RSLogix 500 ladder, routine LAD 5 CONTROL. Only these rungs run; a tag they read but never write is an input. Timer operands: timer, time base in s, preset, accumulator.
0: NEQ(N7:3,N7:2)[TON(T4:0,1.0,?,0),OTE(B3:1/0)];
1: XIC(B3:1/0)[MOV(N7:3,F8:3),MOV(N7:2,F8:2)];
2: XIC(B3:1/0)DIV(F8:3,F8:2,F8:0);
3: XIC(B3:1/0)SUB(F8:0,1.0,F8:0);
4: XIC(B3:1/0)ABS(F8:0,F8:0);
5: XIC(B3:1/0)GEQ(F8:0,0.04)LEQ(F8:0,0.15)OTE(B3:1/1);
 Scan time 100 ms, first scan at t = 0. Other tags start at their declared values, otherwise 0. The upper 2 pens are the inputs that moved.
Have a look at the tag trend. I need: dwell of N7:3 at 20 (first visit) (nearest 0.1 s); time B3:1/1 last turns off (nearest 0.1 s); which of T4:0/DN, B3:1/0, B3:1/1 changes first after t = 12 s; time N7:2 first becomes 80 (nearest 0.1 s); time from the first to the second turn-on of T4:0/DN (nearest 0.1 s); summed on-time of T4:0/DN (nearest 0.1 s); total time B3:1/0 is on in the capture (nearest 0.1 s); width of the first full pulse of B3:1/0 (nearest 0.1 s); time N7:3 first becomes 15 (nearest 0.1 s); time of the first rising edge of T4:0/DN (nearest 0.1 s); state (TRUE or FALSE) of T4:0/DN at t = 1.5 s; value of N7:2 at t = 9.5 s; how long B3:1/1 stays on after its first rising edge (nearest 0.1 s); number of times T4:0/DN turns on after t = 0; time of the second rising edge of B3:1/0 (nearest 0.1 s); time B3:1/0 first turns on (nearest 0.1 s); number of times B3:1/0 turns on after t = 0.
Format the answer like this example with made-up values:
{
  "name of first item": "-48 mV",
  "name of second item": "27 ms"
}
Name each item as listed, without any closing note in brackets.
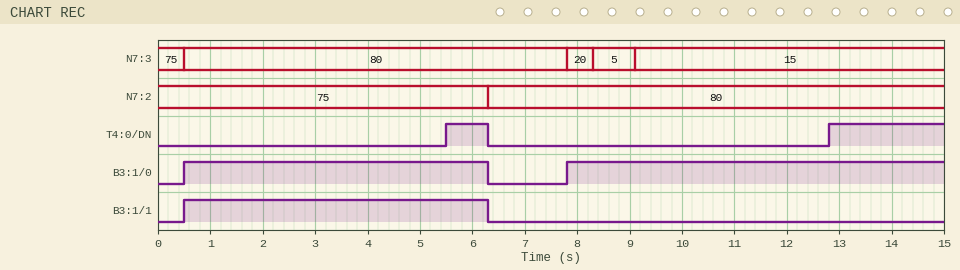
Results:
{
  "dwell of N7:3 at 20 (first visit)": "0.5 s",
  "time B3:1/1 last turns off": "6.3 s",
  "which of T4:0/DN, B3:1/0, B3:1/1 changes first after t = 12 s": "T4:0/DN",
  "time N7:2 first becomes 80": "6.3 s",
  "time from the first to the second turn-on of T4:0/DN": "7.3 s",
  "summed on-time of T4:0/DN": "3.0 s",
  "total time B3:1/0 is on in the capture": "13.0 s",
  "width of the first full pulse of B3:1/0": "5.8 s",
  "time N7:3 first becomes 15": "9.1 s",
  "time of the first rising edge of T4:0/DN": "5.5 s",
  "state (TRUE or FALSE) of T4:0/DN at t = 1.5 s": "FALSE",
  "value of N7:2 at t = 9.5 s": "80",
  "how long B3:1/1 stays on after its first rising edge": "5.8 s",
  "number of times T4:0/DN turns on after t = 0": "2",
  "time of the second rising edge of B3:1/0": "7.8 s",
  "time B3:1/0 first turns on": "0.5 s",
  "number of times B3:1/0 turns on after t = 0": "2"
}
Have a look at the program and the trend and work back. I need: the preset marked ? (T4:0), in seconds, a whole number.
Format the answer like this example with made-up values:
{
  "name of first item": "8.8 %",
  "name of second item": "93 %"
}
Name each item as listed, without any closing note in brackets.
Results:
{
  "the preset marked ? (T4:0), in seconds, a whole number": "5 s"
}
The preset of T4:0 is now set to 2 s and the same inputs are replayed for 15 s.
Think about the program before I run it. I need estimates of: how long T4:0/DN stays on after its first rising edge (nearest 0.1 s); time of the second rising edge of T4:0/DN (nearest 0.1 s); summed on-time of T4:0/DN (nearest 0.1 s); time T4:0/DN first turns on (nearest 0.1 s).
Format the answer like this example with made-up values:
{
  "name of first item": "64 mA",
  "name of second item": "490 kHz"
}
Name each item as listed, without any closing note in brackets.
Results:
{
  "how long T4:0/DN stays on after its first rising edge": "3.8 s",
  "time of the second rising edge of T4:0/DN": "9.8 s",
  "summed on-time of T4:0/DN": "9.0 s",
  "time T4:0/DN first turns on": "2.5 s"
}
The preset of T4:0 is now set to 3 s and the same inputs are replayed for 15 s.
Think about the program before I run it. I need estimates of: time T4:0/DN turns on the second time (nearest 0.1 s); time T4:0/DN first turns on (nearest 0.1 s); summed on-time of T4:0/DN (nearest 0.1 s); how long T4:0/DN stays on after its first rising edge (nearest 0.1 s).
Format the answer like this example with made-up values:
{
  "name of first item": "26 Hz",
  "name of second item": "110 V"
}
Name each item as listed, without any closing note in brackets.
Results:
{
  "time T4:0/DN turns on the second time": "10.8 s",
  "time T4:0/DN first turns on": "3.5 s",
  "summed on-time of T4:0/DN": "7.0 s",
  "how long T4:0/DN stays on after its first rising edge": "2.8 s"
}
